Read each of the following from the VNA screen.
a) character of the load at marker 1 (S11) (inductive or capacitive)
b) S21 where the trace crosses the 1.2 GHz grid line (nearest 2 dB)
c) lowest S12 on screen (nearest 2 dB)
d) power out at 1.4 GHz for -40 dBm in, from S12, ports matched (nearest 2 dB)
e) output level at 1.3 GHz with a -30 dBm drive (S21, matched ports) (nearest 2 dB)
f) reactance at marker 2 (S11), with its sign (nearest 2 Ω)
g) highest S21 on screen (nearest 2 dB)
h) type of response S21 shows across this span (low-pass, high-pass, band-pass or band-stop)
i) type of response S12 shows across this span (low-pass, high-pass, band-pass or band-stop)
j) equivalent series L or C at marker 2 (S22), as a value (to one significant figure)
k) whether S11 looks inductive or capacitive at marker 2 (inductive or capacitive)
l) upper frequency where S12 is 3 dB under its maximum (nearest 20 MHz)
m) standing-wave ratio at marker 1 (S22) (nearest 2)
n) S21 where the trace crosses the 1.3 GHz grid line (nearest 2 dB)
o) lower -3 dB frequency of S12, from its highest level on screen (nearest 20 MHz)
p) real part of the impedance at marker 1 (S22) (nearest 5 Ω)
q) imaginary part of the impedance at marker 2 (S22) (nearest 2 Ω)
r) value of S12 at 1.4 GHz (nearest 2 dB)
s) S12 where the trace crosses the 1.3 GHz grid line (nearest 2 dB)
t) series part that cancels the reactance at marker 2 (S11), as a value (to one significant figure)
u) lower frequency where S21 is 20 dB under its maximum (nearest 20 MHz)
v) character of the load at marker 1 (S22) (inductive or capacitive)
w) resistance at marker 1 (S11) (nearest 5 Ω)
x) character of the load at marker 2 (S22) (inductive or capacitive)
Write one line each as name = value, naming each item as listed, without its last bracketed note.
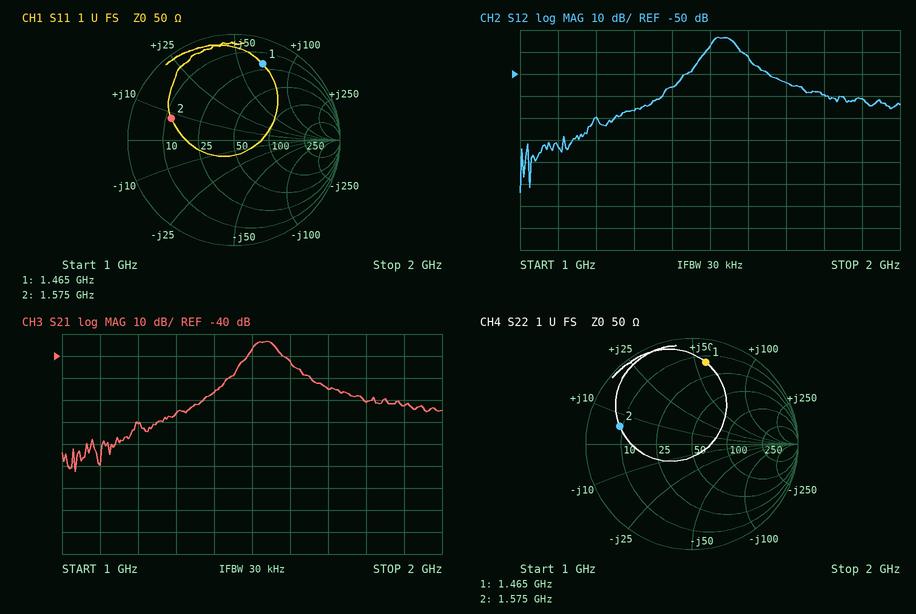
character of the load at marker 1 (S11) = inductive
S21 where the trace crosses the 1.2 GHz grid line = -70 dB
lowest S12 on screen = -104 dB
power out at 1.4 GHz for -40 dBm in, from S12, ports matched = -96 dBm
output level at 1.3 GHz with a -30 dBm drive (S21, matched ports) = -96 dBm
reactance at marker 2 (S11), with its sign = +8 Ω
highest S21 on screen = -34 dB
type of response S21 shows across this span = band-pass
type of response S12 shows across this span = band-pass
equivalent series L or C at marker 2 (S22), as a value = 600 pH
whether S11 looks inductive or capacitive at marker 2 = inductive
upper frequency where S12 is 3 dB under its maximum = 1.56 GHz
standing-wave ratio at marker 1 (S22) = 8
S21 where the trace crosses the 1.3 GHz grid line = -66 dB
lower -3 dB frequency of S12, from its highest level on screen = 1.50 GHz
real part of the impedance at marker 1 (S22) = 15 Ω
imaginary part of the impedance at marker 2 (S22) = +6 Ω
value of S12 at 1.4 GHz = -56 dB
S12 where the trace crosses the 1.3 GHz grid line = -66 dB
series part that cancels the reactance at marker 2 (S11), as a value = 10 pF
lower frequency where S21 is 20 dB under its maximum = 1.42 GHz
character of the load at marker 1 (S22) = inductive
resistance at marker 1 (S11) = 20 Ω
character of the load at marker 2 (S22) = inductive
